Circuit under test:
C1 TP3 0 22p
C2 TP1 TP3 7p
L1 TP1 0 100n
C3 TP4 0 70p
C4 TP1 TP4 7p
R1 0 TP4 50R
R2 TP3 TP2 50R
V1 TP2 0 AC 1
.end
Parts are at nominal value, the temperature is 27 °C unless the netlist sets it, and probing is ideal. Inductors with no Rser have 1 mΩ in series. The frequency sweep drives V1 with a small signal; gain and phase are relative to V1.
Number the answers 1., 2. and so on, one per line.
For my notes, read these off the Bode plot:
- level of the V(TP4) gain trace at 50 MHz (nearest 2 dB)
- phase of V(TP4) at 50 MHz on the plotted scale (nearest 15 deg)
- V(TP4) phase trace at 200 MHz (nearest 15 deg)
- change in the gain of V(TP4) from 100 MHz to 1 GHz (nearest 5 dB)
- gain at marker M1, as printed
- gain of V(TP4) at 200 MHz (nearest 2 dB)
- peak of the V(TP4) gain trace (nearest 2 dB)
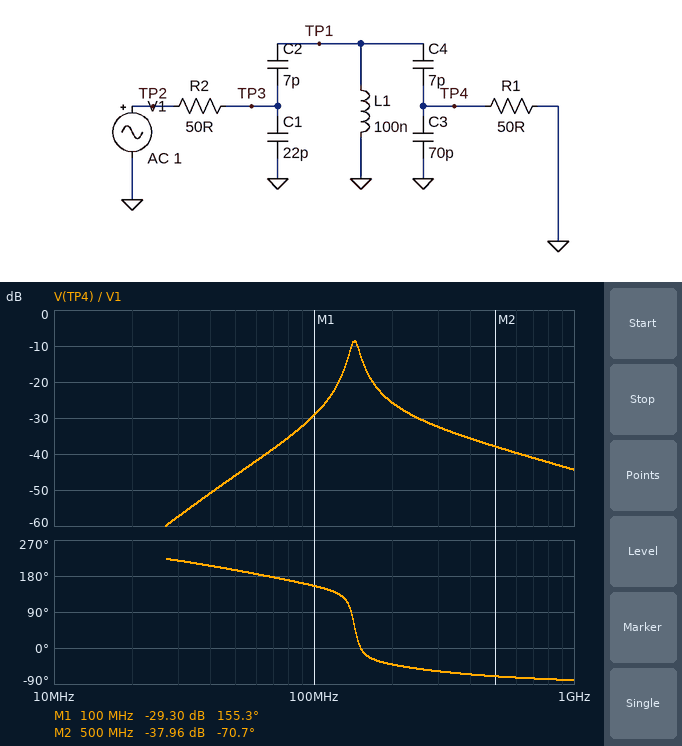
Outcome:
1. -46 dB
2. 195 deg
3. -45 deg
4. -15 dB
5. -29.30 dB
6. -26 dB
7. -8 dB
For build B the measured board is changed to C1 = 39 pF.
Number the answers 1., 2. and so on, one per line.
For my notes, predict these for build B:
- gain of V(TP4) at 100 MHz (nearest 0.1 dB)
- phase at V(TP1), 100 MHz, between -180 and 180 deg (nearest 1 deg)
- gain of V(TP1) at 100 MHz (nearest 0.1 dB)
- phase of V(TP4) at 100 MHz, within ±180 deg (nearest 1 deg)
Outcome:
1. -31.5 dB
2. 121 deg
3. -10.0 dB
4. 144 deg
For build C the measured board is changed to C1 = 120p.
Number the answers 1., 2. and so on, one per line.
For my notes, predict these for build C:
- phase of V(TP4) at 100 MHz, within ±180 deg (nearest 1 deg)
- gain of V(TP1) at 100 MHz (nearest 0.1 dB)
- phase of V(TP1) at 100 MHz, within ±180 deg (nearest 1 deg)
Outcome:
1. 125 deg
2. -17.1 dB
3. 103 deg
